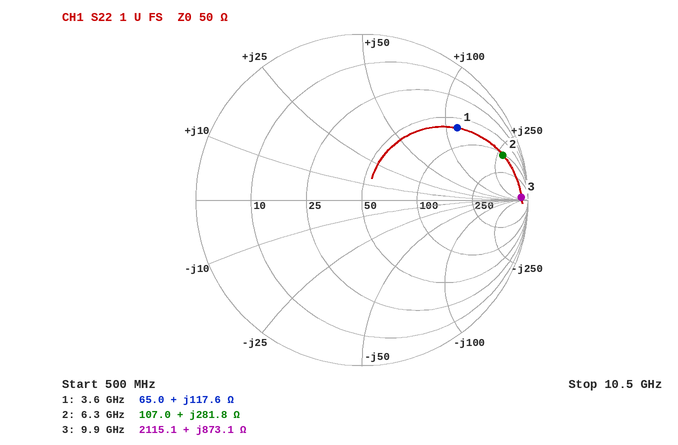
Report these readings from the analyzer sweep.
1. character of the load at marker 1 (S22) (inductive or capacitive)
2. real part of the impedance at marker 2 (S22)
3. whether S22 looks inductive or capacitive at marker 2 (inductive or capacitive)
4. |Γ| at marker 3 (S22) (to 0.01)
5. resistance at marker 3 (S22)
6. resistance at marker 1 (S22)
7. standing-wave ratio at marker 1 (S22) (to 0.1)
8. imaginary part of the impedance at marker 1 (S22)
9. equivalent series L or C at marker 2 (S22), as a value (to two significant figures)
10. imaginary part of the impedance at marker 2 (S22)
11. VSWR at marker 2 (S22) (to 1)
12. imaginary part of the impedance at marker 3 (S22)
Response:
inductive
107.0 Ω
inductive
0.96
2115.1 Ω
65.0 Ω
6.2
+117.6 Ω
7.1 nH
+281.8 Ω
17
+873.1 Ω
